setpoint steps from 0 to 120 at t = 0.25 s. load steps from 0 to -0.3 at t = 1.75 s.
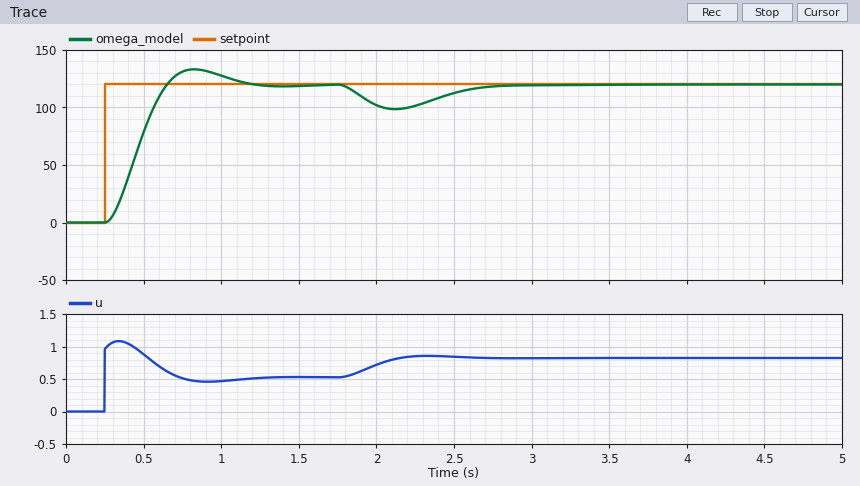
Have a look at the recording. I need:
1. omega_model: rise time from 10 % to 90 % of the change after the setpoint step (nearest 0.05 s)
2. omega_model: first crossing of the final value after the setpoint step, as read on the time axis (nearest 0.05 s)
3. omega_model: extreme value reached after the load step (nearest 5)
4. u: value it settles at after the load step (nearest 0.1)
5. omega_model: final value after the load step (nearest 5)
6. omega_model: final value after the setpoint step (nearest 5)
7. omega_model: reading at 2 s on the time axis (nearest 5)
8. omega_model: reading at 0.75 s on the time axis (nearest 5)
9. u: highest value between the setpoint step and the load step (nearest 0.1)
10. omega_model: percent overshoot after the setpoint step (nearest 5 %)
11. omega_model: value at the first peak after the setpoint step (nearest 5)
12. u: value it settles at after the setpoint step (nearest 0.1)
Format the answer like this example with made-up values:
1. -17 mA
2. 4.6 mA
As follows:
1. 0.25 s
2. 0.65 s
3. 100
4. 0.8
5. 120
6. 120
7. 100
8. 130
9. 1.1
10. 10 %
11. 135
12. 0.5
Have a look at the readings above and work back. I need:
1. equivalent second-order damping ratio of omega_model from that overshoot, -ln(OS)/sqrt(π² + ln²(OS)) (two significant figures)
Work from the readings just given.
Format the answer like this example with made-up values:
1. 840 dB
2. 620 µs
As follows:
1. 0.59
